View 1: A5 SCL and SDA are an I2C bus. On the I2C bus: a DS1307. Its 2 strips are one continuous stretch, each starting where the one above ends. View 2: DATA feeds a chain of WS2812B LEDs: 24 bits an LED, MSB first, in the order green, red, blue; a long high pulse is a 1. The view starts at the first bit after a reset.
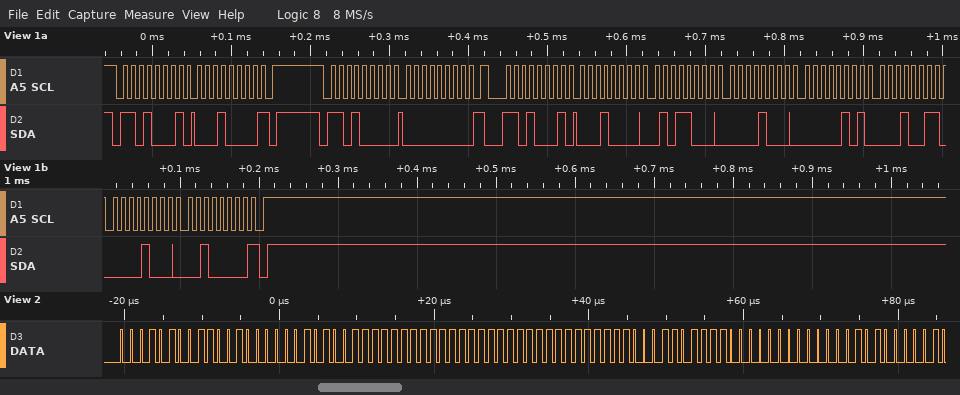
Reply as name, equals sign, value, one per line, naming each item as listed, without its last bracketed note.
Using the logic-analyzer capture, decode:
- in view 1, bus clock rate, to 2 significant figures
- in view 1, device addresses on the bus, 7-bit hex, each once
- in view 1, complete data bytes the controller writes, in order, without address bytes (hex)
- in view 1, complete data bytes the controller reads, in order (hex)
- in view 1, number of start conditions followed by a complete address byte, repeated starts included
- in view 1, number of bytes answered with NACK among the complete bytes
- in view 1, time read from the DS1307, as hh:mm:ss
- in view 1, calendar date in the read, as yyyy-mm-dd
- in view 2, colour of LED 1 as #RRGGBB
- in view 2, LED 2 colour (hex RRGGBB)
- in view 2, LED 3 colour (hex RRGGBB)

in view 1, bus clock rate, to 2 significant figures = 100 kHz
in view 1, device addresses on the bus, 7-bit hex, each once = 0x68
in view 1, complete data bytes the controller writes, in order, without address bytes = 00
in view 1, complete data bytes the controller reads, in order = 10 10 58 08 05 13 08 20
in view 1, number of start conditions followed by a complete address byte, repeated starts included = 3
in view 1, number of bytes answered with NACK among the complete bytes = 2
in view 1, time read from the DS1307, as hh:mm:ss = 08:58:10
in view 1, calendar date in the read, as yyyy-mm-dd = 2020-08-13
in view 2, colour of LED 1 as #RRGGBB = #C81414
in view 2, LED 2 colour = #FFFFFF
in view 2, LED 3 colour = #DEF800
